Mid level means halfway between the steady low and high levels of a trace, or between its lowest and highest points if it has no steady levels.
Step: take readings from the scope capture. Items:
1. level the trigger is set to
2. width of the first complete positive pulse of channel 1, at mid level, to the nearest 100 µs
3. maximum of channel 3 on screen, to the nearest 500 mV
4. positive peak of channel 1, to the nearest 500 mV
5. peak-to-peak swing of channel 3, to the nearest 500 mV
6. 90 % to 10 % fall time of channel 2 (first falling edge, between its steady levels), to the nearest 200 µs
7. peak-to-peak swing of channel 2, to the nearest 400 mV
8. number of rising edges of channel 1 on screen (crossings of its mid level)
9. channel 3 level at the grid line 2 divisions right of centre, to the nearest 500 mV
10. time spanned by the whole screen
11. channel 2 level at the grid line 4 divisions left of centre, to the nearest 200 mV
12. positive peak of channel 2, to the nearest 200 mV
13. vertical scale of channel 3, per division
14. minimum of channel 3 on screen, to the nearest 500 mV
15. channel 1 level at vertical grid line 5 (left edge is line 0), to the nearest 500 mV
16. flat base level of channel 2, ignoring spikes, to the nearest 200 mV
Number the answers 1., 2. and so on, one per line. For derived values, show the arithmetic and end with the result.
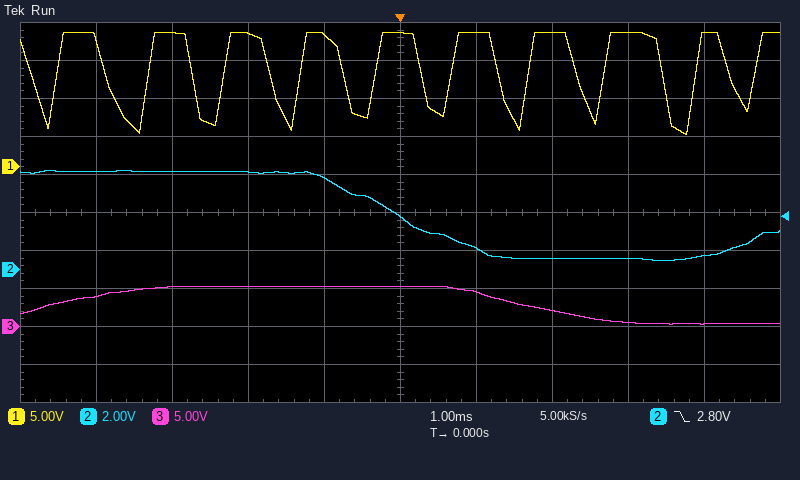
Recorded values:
1. 2.80 V
2. 700 µs
3. 5.5 V
4. 17.5 V
5. 5.5 V − (500 mV) = 5.0 V
6. 2.0 ms
7. 4.8 V
8. 10
9. 2.0 V
10. 10 ms
11. 5.2 V
12. 5.2 V
13. 5 V
14. 500 mV
15. 17.5 V
16. 600 mV
